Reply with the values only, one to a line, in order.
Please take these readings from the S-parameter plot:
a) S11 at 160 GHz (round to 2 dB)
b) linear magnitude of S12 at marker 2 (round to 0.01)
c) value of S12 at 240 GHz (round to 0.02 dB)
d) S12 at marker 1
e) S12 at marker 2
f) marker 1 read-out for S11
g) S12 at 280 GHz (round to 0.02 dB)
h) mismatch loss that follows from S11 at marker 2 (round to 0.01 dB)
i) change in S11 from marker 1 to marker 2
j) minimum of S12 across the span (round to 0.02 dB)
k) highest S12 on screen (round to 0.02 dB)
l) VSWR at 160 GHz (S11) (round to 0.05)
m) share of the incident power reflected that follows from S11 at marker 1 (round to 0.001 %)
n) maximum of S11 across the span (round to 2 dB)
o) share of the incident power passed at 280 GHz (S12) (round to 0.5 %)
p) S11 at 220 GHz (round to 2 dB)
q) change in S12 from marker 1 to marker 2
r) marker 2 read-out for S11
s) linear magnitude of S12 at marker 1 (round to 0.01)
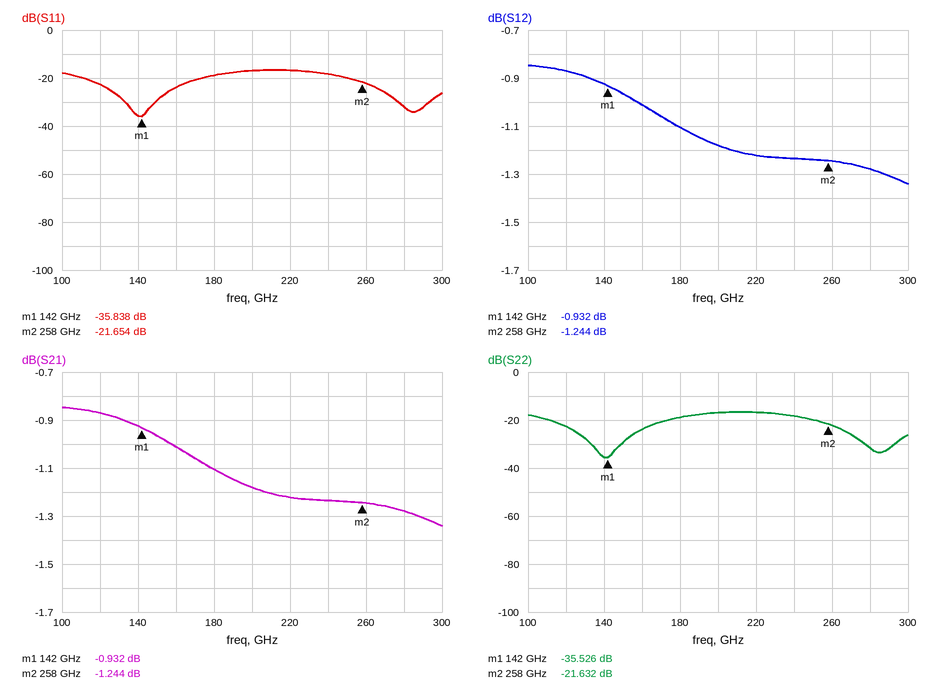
-24 dB
0.87
-1.24 dB
-0.932 dB
-1.244 dB
-35.838 dB
-1.28 dB
0.03 dB
14.184 dB
-1.34 dB
-0.84 dB
1.15
0.026 %
-16 dB
74.5 %
-16 dB
-0.312 dB
-21.654 dB
0.90
